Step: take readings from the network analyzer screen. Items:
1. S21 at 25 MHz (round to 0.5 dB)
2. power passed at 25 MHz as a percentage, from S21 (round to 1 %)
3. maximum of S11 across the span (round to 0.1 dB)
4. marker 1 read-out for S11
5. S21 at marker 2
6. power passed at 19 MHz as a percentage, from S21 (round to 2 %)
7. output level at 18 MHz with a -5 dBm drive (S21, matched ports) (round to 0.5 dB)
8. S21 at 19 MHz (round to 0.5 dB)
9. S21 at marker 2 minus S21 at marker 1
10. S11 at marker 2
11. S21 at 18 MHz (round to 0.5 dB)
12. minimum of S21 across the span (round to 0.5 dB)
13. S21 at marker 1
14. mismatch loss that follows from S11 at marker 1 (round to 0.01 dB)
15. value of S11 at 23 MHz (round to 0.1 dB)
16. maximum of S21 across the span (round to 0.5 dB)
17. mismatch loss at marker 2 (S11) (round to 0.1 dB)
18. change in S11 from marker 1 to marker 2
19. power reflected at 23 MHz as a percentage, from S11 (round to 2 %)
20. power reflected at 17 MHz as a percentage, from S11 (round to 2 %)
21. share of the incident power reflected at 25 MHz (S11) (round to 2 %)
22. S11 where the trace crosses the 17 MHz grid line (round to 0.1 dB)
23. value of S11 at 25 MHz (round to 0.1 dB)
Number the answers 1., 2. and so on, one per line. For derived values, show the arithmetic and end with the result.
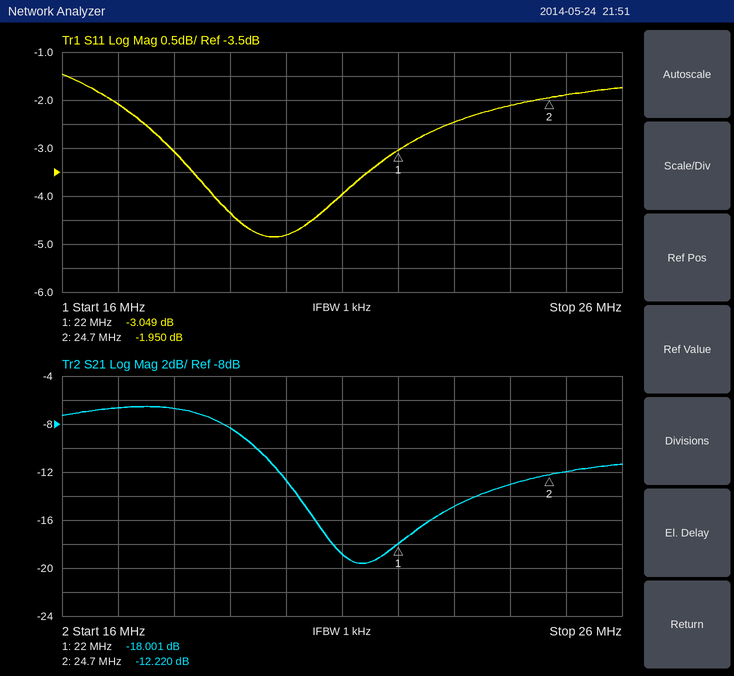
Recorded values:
1. -12.0 dB
2. 10^(-12/10) ≈ 6 %
3. -1.5 dB
4. -3.049 dB
5. -12.220 dB
6. 10^(-8.5/10) ≈ 14 %
7. -5 dBm + (-6.5 dB) = -11.5 dBm
8. -8.5 dB
9. -12.22 − (-18.001) = 5.781 dB
10. -1.950 dB
11. -6.5 dB
12. -19.5 dB
13. -18.001 dB
14. −10 log10(1 − 10^(-3.049/10)) ≈ 2.97 dB
15. -2.5 dB
16. -6.5 dB
17. −10 log10(1 − 10^(-1.95/10)) ≈ 4.4 dB
18. -1.95 − (-3.049) = 1.099 dB
19. 10^(-2.5/10) ≈ 56 %
20. 10^(-2.1/10) ≈ 62 %
21. 10^(-1.9/10) ≈ 64.6 %, so 64 % to the nearest 2 %
22. -2.1 dB
23. -1.9 dB
